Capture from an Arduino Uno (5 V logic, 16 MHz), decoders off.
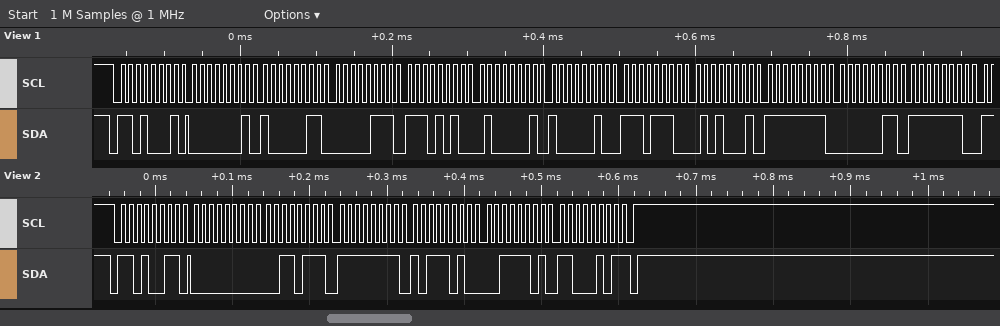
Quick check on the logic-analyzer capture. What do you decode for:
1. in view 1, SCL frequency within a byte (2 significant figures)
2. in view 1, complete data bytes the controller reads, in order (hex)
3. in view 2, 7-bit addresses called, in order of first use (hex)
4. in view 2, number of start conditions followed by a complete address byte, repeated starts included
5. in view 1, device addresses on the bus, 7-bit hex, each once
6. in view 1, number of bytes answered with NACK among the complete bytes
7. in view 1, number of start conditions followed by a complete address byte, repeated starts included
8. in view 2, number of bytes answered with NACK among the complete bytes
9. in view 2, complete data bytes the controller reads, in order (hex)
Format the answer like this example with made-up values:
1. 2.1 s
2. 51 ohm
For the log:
1. 100 kHz
2. 01 83 07 EA 41 82 EE 51 FF 03 FE
3. 0x69
4. 1
5. 0x68
6. 0
7. 1
8. 1
9. 00 37 FF BA 3D C5
